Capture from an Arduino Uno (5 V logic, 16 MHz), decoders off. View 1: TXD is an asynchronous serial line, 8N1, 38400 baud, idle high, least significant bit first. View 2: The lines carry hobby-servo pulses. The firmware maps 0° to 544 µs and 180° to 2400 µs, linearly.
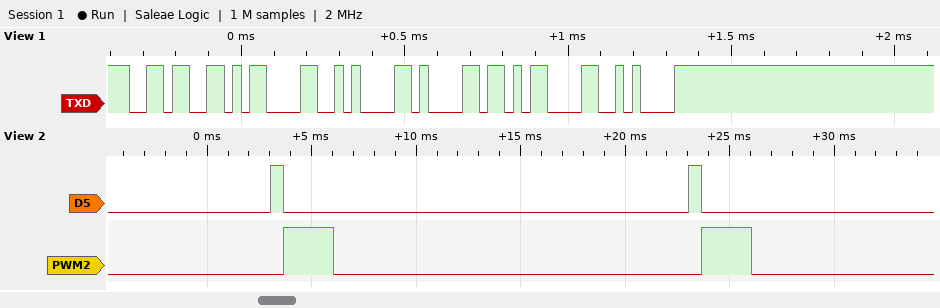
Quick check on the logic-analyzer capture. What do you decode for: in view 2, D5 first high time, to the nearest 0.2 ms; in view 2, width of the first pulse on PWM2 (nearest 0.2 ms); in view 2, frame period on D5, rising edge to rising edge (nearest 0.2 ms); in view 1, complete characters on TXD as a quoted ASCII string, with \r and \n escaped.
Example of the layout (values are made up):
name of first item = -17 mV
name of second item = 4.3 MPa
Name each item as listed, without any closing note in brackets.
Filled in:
in view 2, D5 first high time, to the nearest 0.2 ms = 0.6 ms
in view 2, width of the first pulse on PWM2 = 2.4 ms
in view 2, frame period on D5, rising edge to rising edge = 20.0 ms
in view 1, complete characters on TXD as a quoted ASCII string, with \r and \n escaped = "6\r\na\r\n"
